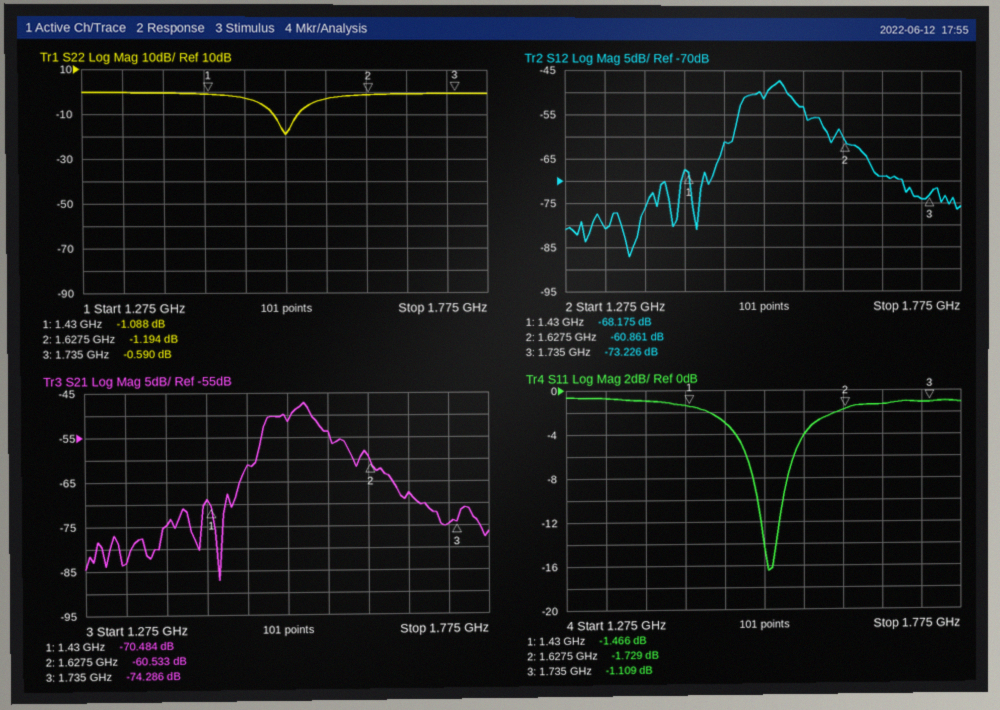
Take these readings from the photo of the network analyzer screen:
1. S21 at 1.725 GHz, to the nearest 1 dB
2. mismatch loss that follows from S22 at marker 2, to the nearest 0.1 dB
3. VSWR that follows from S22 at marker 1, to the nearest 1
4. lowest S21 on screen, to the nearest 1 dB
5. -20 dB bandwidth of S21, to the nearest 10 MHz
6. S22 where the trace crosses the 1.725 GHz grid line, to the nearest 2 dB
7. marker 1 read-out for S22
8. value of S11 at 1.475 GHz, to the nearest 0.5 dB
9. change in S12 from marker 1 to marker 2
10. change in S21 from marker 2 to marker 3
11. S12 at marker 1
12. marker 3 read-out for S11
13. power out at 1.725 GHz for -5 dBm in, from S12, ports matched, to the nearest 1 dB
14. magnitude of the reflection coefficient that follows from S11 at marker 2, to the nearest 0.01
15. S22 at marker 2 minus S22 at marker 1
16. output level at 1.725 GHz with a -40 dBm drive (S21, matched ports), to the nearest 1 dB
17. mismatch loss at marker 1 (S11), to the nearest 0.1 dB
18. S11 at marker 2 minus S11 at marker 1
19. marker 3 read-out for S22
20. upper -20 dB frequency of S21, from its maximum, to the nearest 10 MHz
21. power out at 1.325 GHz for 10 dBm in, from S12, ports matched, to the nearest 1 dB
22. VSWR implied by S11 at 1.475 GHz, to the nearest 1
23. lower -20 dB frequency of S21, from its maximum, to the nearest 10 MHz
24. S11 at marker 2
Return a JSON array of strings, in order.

["-75 dB", "6.2 dB", "16", "-87 dB", "200 MHz", "0 dB", "-1.088 dB", "-3.0 dB", "7.314 dB", "-13.753 dB", "-68.175 dB", "-1.109 dB", "-79 dBm", "0.82", "-0.106 dB", "-115 dBm", "5.4 dB", "-0.263 dB", "-0.590 dB", "1.66 GHz", "-71 dBm", "6", "1.46 GHz", "-1.729 dB"]
